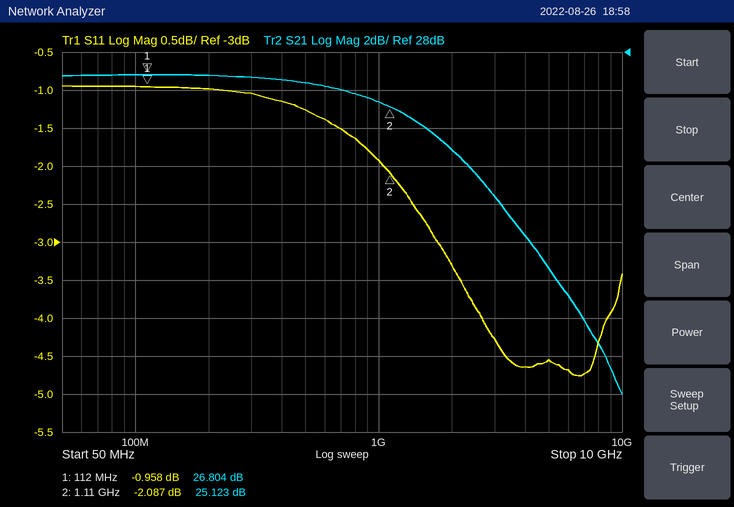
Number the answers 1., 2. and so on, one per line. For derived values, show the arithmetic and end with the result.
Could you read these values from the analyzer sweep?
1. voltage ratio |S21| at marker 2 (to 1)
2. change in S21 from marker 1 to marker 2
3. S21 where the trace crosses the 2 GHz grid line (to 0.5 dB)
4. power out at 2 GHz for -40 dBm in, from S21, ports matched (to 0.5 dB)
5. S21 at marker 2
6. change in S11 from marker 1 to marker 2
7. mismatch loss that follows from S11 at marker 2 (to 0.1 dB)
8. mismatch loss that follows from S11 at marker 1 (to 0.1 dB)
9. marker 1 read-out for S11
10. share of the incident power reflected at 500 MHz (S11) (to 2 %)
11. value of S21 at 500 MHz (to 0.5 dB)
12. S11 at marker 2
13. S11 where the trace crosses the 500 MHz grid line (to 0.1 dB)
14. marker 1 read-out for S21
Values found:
1. 10^(25.123/20) ≈ 18
2. 25.123 − (26.804) = -1.681 dB
3. 23.0 dB
4. -40 dBm + (23.0 dB) = -17.0 dBm
5. 25.123 dB
6. -2.087 − (-0.958) = -1.129 dB
7. −10 log10(1 − 10^(-2.087/10)) ≈ 4.2 dB
8. −10 log10(1 − 10^(-0.958/10)) ≈ 7.0 dB
9. -0.958 dB
10. 10^(-1.3/10) ≈ 74 %
11. 26.5 dB
12. -2.087 dB
13. -1.3 dB
14. 26.804 dB
